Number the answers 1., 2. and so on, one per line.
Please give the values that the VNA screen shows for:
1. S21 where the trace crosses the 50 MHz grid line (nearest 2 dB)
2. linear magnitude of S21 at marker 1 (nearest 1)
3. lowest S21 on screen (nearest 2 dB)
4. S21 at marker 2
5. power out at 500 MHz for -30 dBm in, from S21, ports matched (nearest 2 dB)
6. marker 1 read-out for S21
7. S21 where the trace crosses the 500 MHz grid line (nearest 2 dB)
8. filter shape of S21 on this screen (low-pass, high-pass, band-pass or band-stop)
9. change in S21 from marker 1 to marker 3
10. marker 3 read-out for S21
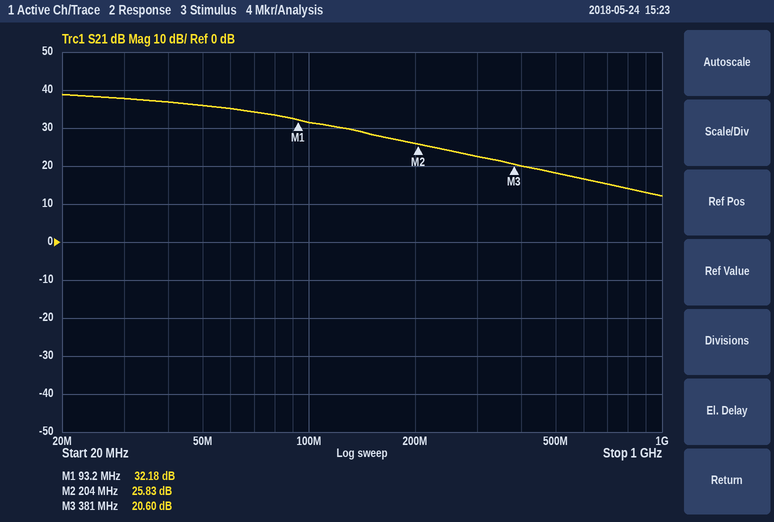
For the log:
1. 36 dB
2. 41
3. 12 dB
4. 25.83 dB
5. -12 dBm
6. 32.18 dB
7. 18 dB
8. low-pass
9. -11.58 dB
10. 20.60 dB
